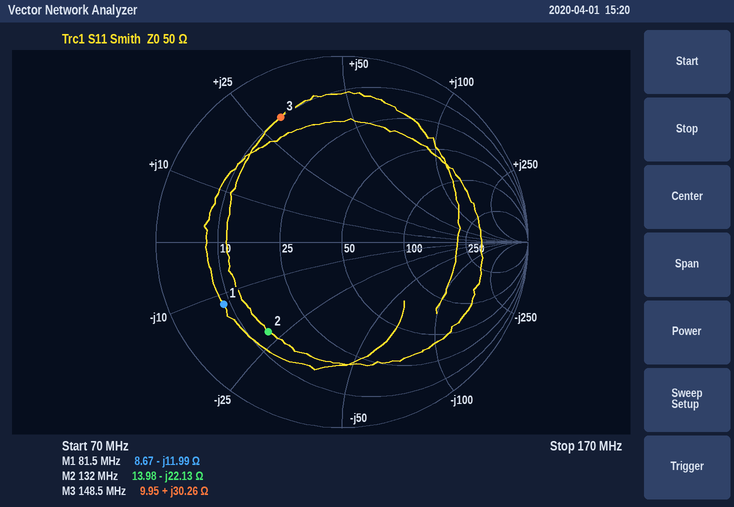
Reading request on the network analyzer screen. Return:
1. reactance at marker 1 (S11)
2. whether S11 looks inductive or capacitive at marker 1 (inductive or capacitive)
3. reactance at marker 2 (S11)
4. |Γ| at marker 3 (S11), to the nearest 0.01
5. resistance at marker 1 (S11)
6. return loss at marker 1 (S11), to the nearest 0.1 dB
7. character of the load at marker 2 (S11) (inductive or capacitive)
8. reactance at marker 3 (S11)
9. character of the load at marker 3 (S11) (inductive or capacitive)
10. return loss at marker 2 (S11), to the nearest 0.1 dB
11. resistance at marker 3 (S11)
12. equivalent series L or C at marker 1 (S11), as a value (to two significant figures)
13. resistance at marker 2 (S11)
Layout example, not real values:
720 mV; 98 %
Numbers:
-11.99 Ω; capacitive; -22.13 Ω; 0.75; 8.67 Ω; 2.9 dB; capacitive; +30.26 Ω; inductive; 4.1 dB; 9.95 Ω; 160 pF; 13.98 Ω
